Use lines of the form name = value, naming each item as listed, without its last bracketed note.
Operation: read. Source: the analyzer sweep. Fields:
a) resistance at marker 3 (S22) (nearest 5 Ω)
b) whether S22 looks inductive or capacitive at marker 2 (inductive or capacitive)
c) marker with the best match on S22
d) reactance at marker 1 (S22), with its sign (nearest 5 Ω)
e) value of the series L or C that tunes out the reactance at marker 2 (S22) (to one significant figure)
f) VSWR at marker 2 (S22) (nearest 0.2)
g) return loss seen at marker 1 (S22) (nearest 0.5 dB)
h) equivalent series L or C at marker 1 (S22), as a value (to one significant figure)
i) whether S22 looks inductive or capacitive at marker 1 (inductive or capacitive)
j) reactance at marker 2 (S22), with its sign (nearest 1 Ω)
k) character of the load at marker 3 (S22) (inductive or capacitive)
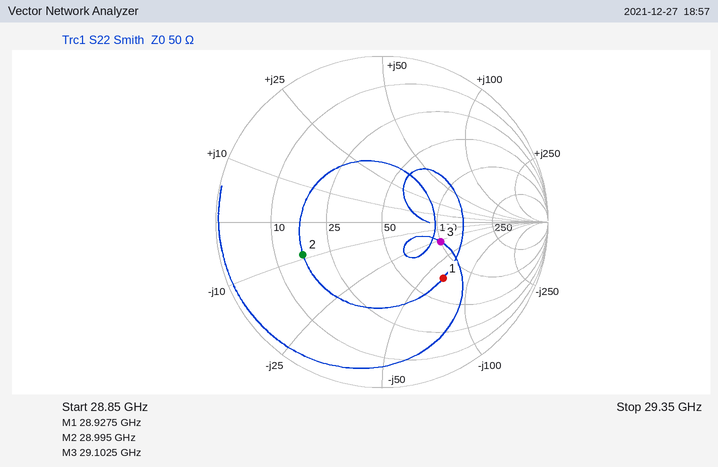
resistance at marker 3 (S22) = 100 Ω
whether S22 looks inductive or capacitive at marker 2 = capacitive
marker with the best match on S22 = marker 3
reactance at marker 1 (S22), with its sign = -65 Ω
value of the series L or C that tunes out the reactance at marker 2 (S22) = 50 pH
VSWR at marker 2 (S22) = 3.2
return loss seen at marker 1 (S22) = 6.0 dB
equivalent series L or C at marker 1 (S22), as a value = 80 fF
whether S22 looks inductive or capacitive at marker 1 = capacitive
reactance at marker 2 (S22), with its sign = -9 Ω
character of the load at marker 3 (S22) = capacitive
